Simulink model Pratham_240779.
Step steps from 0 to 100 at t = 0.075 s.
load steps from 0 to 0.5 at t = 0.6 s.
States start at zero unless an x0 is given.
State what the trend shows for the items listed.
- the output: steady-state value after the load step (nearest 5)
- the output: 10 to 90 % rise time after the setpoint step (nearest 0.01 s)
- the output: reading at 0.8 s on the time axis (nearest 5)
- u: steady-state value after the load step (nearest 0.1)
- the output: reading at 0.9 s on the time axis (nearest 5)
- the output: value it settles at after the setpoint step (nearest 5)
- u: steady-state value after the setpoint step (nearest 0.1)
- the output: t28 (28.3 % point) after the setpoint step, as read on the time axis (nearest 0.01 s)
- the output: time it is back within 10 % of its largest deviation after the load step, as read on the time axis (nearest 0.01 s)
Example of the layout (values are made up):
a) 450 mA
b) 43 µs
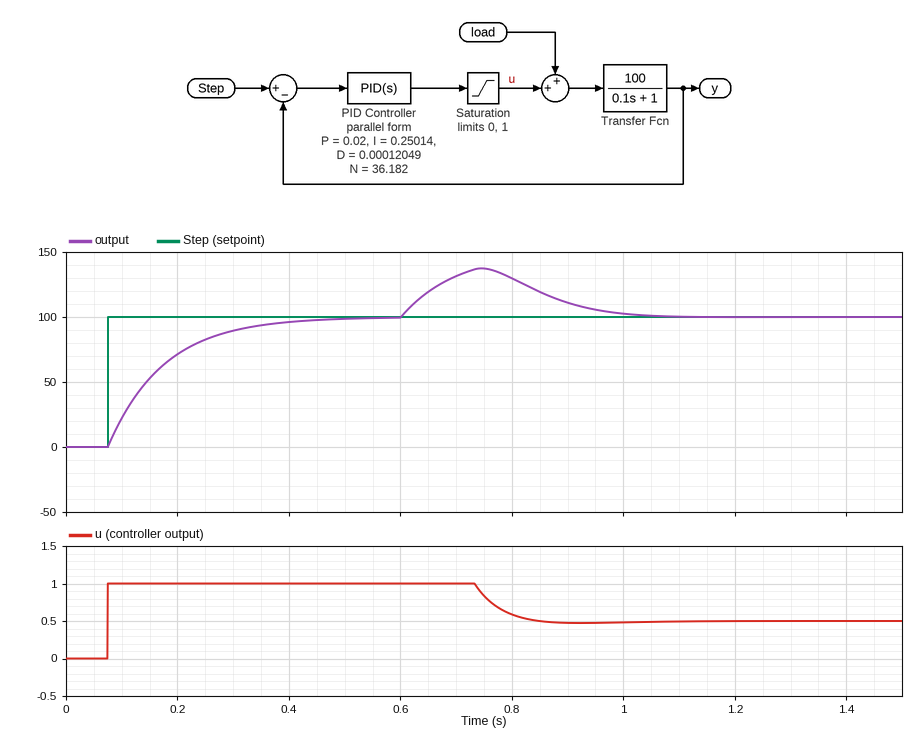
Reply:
a) 100
b) 0.22 s
c) 130
d) 0.5
e) 110
f) 100
g) 1.0
h) 0.11 s
i) 0.98 s
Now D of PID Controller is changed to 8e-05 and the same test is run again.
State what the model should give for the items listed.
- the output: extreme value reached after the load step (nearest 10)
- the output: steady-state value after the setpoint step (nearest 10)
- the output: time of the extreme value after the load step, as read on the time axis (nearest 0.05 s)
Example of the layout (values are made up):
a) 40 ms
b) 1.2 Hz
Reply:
a) 140
b) 100
c) 0.75 s
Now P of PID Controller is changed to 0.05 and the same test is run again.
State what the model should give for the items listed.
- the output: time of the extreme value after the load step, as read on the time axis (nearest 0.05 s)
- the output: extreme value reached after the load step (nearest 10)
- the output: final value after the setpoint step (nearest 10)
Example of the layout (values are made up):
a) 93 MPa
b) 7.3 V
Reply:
a) 0.70 s
b) 130
c) 100
